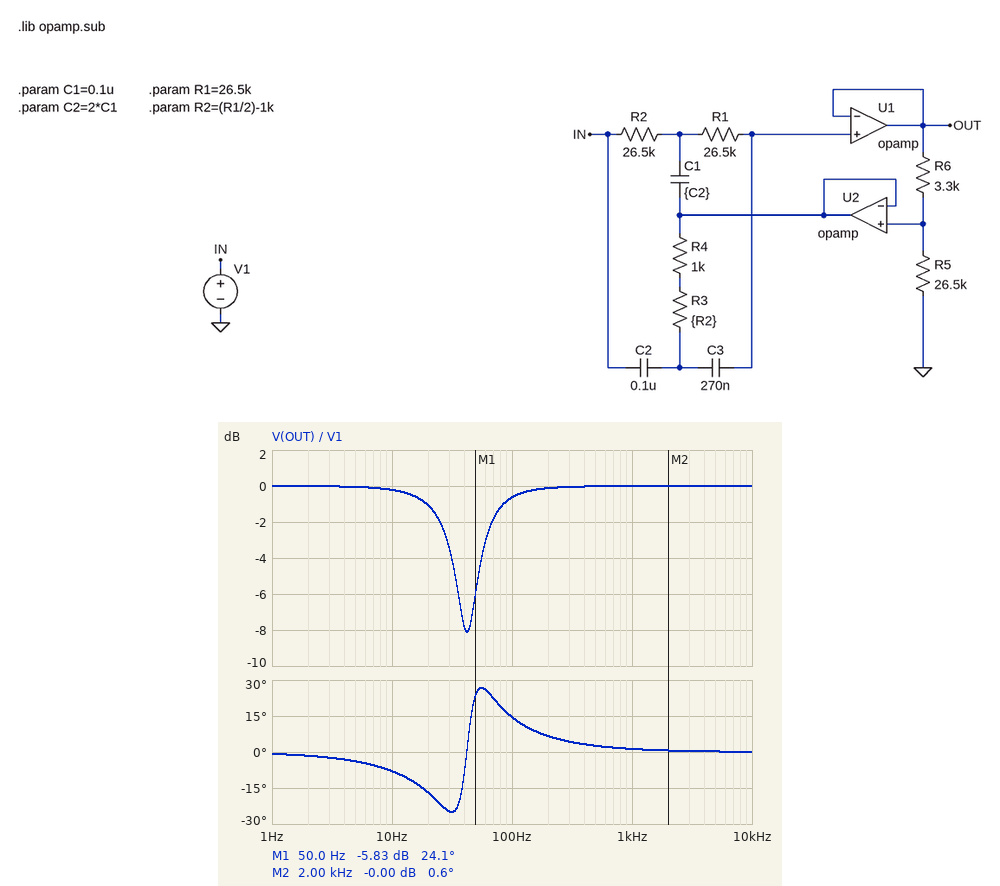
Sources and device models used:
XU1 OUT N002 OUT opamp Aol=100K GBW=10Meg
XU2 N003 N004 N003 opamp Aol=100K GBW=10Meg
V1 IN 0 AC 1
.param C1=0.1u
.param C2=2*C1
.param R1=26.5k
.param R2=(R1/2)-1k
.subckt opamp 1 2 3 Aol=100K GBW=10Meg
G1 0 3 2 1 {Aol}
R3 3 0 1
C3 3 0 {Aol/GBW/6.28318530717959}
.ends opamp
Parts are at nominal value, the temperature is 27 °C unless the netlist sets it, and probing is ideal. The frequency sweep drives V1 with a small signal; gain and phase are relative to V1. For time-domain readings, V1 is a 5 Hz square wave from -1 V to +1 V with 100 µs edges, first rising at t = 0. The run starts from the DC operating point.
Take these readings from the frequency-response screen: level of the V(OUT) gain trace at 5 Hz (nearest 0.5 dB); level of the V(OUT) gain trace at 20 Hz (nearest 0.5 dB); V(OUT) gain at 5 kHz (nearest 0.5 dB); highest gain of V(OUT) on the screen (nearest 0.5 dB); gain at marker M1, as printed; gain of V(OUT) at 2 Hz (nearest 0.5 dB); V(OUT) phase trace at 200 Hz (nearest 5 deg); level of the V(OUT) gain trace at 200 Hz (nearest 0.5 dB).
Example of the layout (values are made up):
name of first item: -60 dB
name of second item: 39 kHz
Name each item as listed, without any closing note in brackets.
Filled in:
level of the V(OUT) gain trace at 5 Hz: 0 dB
level of the V(OUT) gain trace at 20 Hz: -1.0 dB
V(OUT) gain at 5 kHz: 0 dB
highest gain of V(OUT) on the screen: 0 dB
gain at marker M1, as printed: -5.83 dB
gain of V(OUT) at 2 Hz: 0 dB
V(OUT) phase trace at 200 Hz: 5 deg
level of the V(OUT) gain trace at 200 Hz: 0 dB
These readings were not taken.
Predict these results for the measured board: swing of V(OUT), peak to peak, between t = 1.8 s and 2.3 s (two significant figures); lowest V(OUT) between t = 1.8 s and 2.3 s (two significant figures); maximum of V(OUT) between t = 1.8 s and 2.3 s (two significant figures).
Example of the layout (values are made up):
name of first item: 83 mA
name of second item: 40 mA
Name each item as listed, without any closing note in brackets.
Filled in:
swing of V(OUT), peak to peak, between t = 1.8 s and 2.3 s: 2.2 V
lowest V(OUT) between t = 1.8 s and 2.3 s: -1.1 V
maximum of V(OUT) between t = 1.8 s and 2.3 s: 1.1 V
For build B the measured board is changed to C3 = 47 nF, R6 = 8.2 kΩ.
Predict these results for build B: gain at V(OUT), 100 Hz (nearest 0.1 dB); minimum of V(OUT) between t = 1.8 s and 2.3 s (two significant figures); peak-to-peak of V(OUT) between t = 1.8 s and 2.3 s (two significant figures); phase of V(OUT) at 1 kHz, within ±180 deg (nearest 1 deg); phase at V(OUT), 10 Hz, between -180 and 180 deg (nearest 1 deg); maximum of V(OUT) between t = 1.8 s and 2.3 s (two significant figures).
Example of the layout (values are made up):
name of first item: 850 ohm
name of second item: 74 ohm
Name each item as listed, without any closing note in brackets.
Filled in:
gain at V(OUT), 100 Hz: -5.6 dB
minimum of V(OUT) between t = 1.8 s and 2.3 s: -1.3 V
peak-to-peak of V(OUT) between t = 1.8 s and 2.3 s: 2.6 V
phase of V(OUT) at 1 kHz, within ±180 deg: 4 deg
phase at V(OUT), 10 Hz, between -180 and 180 deg: -7 deg
maximum of V(OUT) between t = 1.8 s and 2.3 s: 1.3 V
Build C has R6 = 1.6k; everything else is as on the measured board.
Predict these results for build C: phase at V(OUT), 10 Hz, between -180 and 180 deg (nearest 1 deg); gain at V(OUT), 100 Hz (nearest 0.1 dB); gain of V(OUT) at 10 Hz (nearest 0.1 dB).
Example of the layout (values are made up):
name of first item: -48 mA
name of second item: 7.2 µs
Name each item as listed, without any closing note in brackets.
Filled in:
phase at V(OUT), 10 Hz, between -180 and 180 deg: -4 deg
gain at V(OUT), 100 Hz: -0.3 dB
gain of V(OUT) at 10 Hz: -0.1 dB
